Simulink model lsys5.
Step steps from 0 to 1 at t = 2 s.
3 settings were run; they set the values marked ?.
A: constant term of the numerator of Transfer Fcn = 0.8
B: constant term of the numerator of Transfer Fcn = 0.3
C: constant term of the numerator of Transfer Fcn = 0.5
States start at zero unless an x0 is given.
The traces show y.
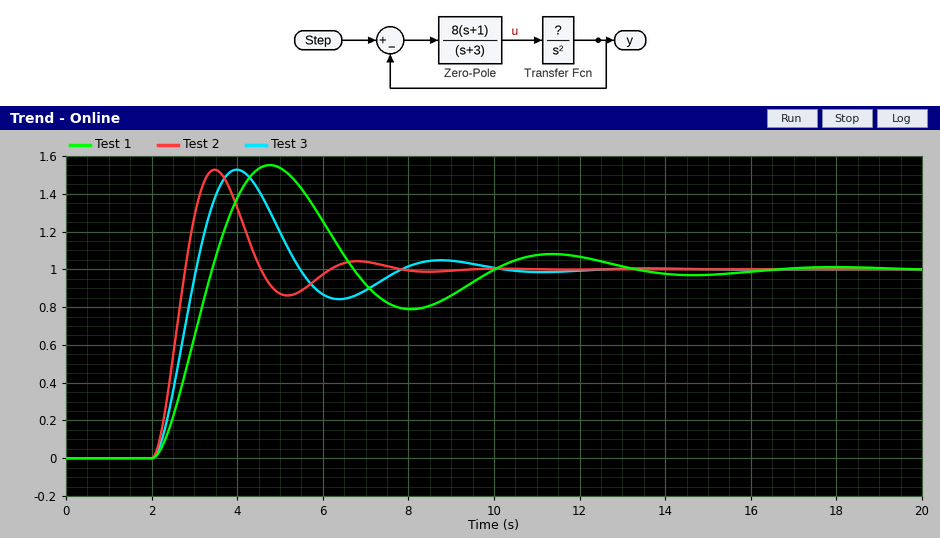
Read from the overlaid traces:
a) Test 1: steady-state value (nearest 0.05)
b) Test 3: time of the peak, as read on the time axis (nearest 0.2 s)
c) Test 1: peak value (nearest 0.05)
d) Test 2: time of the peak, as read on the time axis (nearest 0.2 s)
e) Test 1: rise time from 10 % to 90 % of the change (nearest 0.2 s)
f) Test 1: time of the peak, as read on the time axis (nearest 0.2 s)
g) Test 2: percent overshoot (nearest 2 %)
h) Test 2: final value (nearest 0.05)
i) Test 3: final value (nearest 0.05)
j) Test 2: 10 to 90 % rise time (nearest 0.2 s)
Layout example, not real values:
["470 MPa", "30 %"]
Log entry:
["1.00", "4.0 s", "1.55", "3.4 s", "1.0 s", "4.8 s", "52 %", "1.00", "1.00", "0.6 s"]
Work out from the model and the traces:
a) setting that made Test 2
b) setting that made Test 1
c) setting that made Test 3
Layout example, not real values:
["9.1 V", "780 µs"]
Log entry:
["A", "B", "C"]
